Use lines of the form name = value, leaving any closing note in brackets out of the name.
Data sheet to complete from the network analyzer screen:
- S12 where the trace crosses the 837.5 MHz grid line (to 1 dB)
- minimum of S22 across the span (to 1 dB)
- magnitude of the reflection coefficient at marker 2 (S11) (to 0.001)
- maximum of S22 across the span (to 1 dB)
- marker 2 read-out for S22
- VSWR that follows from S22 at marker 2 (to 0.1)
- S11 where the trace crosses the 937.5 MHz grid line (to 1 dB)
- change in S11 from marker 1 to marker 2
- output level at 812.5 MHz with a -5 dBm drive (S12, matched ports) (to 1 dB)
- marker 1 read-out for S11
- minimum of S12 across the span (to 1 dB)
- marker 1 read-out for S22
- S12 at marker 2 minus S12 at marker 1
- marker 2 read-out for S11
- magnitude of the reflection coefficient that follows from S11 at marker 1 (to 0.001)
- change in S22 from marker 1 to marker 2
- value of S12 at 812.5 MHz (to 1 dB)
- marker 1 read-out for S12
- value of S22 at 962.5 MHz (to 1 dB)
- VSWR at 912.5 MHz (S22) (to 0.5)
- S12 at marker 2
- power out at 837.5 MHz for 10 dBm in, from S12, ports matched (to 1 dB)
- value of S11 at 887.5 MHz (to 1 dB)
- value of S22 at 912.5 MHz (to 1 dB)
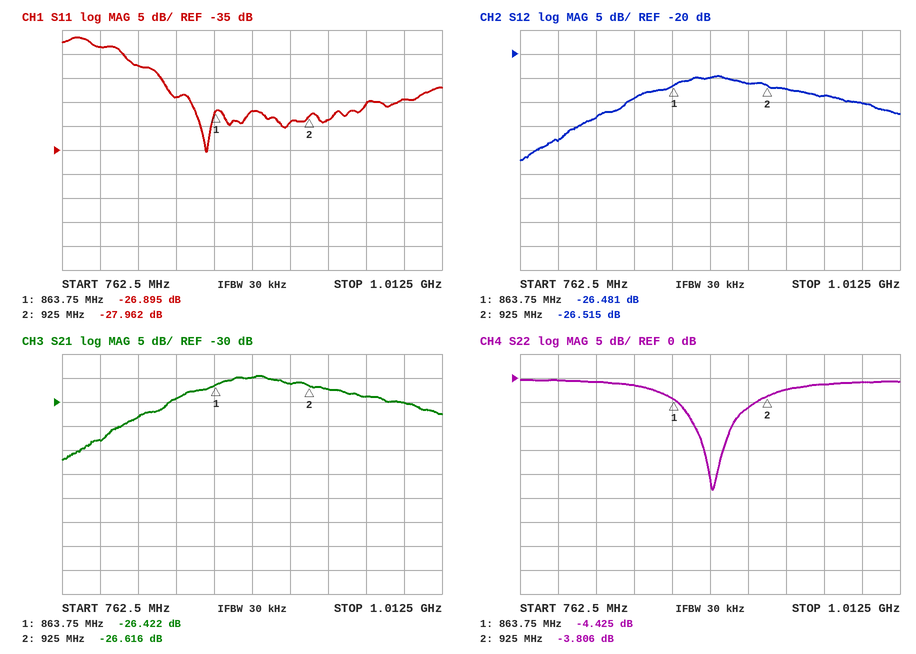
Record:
S12 where the trace crosses the 837.5 MHz grid line = -29 dB
minimum of S22 across the span = -23 dB
magnitude of the reflection coefficient at marker 2 (S11) = 0.040
maximum of S22 across the span = 0 dB
marker 2 read-out for S22 = -3.806 dB
VSWR that follows from S22 at marker 2 = 4.6
S11 where the trace crosses the 937.5 MHz grid line = -29 dB
change in S11 from marker 1 to marker 2 = -1.067 dB
output level at 812.5 MHz with a -5 dBm drive (S12, matched ports) = -38 dBm
marker 1 read-out for S11 = -26.895 dB
minimum of S12 across the span = -42 dB
marker 1 read-out for S22 = -4.425 dB
S12 at marker 2 minus S12 at marker 1 = -0.034 dB
marker 2 read-out for S11 = -27.962 dB
magnitude of the reflection coefficient that follows from S11 at marker 1 = 0.045
change in S22 from marker 1 to marker 2 = 0.619 dB
value of S12 at 812.5 MHz = -33 dB
marker 1 read-out for S12 = -26.481 dB
value of S22 at 962.5 MHz = -1 dB
VSWR at 912.5 MHz (S22) = 3.0
S12 at marker 2 = -26.515 dB
power out at 837.5 MHz for 10 dBm in, from S12, ports matched = -19 dBm
value of S11 at 887.5 MHz = -27 dB
value of S22 at 912.5 MHz = -6 dB
